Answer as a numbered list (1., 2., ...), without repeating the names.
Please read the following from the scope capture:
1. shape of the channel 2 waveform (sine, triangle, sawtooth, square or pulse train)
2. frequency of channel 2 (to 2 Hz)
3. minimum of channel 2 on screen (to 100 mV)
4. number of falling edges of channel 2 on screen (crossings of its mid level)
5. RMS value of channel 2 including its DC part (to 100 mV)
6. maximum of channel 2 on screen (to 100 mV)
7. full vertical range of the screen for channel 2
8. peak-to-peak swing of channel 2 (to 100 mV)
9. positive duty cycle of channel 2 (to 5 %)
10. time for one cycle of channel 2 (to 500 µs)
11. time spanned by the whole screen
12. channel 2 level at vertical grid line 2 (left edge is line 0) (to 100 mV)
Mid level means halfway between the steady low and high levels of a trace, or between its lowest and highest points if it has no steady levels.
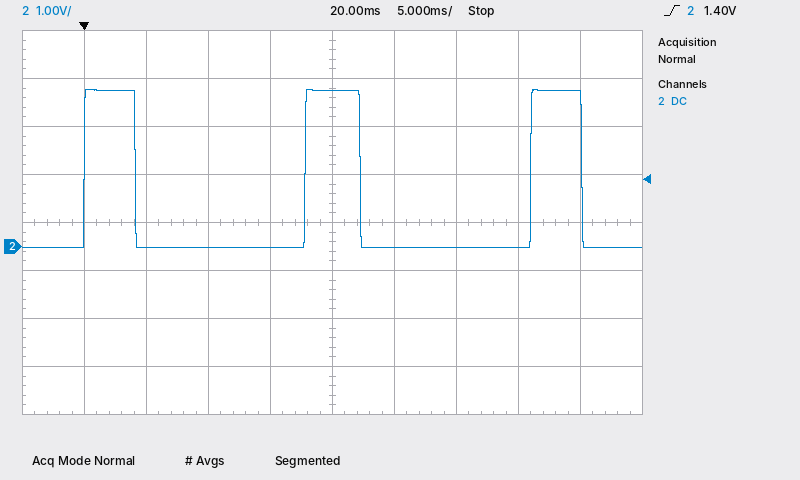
1. pulse train
2. 56 Hz
3. 0.0 V
4. 3
5. 1.6 V
6. 3.3 V
7. 8 V
8. 3.3 V
9. 25 %
10. 18.0 ms
11. 50 ms
12. 0.0 V
